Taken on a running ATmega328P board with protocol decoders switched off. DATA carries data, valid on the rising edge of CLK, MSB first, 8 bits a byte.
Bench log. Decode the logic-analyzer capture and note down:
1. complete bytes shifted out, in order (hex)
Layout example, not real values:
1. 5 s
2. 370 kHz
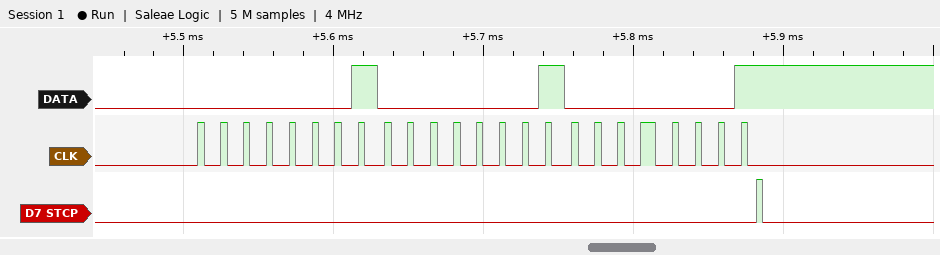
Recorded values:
1. 0x01 0x01 0x01
